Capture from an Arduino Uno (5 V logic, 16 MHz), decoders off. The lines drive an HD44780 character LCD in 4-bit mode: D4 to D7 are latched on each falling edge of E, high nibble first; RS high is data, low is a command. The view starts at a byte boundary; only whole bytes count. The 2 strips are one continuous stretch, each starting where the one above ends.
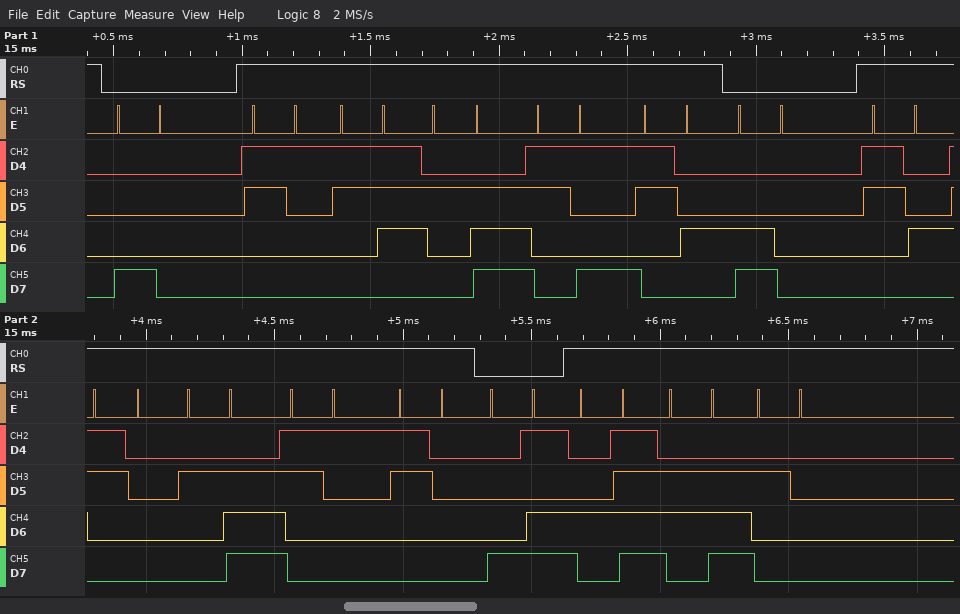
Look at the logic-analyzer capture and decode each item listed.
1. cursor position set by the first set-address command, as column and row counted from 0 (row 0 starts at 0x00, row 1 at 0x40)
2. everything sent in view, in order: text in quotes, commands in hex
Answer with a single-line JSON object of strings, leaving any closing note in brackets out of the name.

{"cursor position set by the first set-address command, as column and row counted from 0": "column 0, row 0", "everything sent in view, in order: text in quotes, commands in hex": "0x80 \"17.94\" 0xC0 \"40.10\" 0x8D \"On \""}
